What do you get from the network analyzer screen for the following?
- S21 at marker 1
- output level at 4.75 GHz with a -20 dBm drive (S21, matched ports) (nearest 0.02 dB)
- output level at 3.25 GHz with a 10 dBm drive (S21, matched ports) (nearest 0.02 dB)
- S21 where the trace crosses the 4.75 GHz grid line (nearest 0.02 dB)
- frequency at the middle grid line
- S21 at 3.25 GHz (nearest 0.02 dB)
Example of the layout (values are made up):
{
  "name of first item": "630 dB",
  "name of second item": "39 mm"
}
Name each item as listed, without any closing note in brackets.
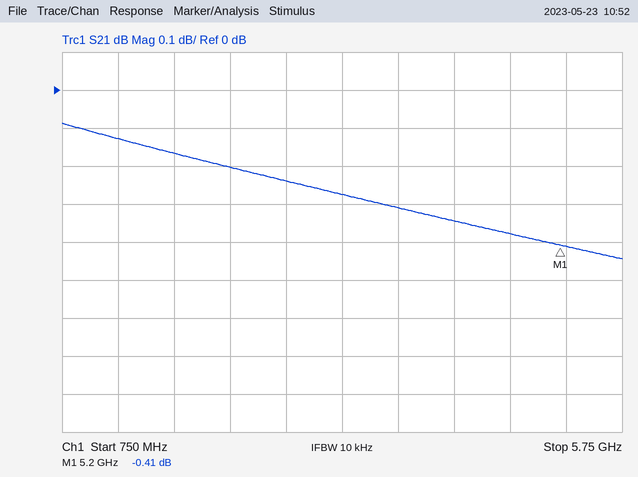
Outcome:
{
  "S21 at marker 1": "-0.41 dB",
  "output level at 4.75 GHz with a -20 dBm drive (S21, matched ports)": "-20.38 dBm",
  "output level at 3.25 GHz with a 10 dBm drive (S21, matched ports)": "9.72 dBm",
  "S21 where the trace crosses the 4.75 GHz grid line": "-0.38 dB",
  "frequency at the middle grid line": "3.25 GHz",
  "S21 at 3.25 GHz": "-0.28 dB"
}
